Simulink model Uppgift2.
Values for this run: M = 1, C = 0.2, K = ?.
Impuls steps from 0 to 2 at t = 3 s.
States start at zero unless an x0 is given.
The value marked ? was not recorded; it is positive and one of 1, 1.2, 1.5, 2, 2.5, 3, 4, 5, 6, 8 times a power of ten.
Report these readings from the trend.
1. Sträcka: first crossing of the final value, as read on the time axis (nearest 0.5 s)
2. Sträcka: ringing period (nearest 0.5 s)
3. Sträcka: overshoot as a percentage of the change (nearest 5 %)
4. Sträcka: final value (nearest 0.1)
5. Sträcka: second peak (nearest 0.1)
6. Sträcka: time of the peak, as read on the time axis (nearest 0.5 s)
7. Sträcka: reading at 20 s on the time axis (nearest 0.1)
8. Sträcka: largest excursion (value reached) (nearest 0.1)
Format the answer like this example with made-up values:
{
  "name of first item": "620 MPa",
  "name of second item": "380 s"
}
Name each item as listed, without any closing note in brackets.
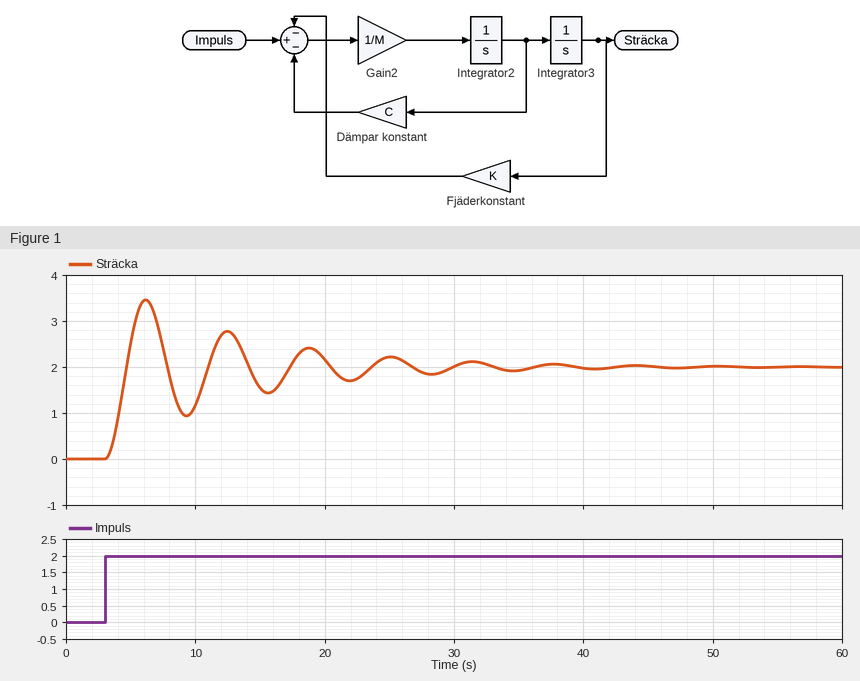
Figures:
{
  "Sträcka: first crossing of the final value, as read on the time axis": "4.5 s",
  "Sträcka: ringing period": "6.5 s",
  "Sträcka: overshoot as a percentage of the change": "75 %",
  "Sträcka: final value": "2.0",
  "Sträcka: second peak": "2.8",
  "Sträcka: time of the peak, as read on the time axis": "6.0 s",
  "Sträcka: reading at 20 s on the time axis": "2.2",
  "Sträcka: largest excursion (value reached)": "3.5"
}
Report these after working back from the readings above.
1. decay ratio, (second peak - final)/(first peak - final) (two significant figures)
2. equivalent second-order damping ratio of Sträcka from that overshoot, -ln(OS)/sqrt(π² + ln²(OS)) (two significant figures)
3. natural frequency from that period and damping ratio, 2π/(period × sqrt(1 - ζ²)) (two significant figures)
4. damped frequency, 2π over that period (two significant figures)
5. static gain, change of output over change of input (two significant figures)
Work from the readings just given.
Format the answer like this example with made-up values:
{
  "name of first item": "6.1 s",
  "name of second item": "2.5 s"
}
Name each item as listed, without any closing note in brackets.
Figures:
{
  "decay ratio, (second peak - final)/(first peak - final)": "0.53",
  "equivalent second-order damping ratio of Sträcka from that overshoot, -ln(OS)/sqrt(π² + ln²(OS))": "0.091",
  "natural frequency from that period and damping ratio, 2π/(period × sqrt(1 - ζ²))": "0.97 rad/s",
  "damped frequency, 2π over that period": "0.97 rad/s",
  "static gain, change of output over change of input": "1.0"
}
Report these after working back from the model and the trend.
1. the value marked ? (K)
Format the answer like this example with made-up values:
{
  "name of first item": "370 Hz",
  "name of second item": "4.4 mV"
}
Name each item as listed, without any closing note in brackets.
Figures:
{
  "the value marked ?": "1"
}
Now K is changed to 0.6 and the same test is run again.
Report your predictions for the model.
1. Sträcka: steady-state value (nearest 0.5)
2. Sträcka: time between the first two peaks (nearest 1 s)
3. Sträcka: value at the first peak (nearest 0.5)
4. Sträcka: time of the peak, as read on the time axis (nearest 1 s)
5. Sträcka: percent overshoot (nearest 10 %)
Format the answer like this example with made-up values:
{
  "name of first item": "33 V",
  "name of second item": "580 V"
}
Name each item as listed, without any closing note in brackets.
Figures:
{
  "Sträcka: steady-state value": "3.5",
  "Sträcka: time between the first two peaks": "8 s",
  "Sträcka: value at the first peak": "5.5",
  "Sträcka: time of the peak, as read on the time axis": "7 s",
  "Sträcka: percent overshoot": "70 %"
}
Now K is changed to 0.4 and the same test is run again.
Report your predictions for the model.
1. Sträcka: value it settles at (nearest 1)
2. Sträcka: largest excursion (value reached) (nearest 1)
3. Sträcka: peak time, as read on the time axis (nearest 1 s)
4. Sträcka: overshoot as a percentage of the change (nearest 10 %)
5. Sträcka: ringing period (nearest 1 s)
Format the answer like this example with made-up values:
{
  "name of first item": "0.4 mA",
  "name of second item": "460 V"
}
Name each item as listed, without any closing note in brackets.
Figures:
{
  "Sträcka: value it settles at": "5",
  "Sträcka: largest excursion (value reached)": "8",
  "Sträcka: peak time, as read on the time axis": "8 s",
  "Sträcka: overshoot as a percentage of the change": "60 %",
  "Sträcka: ringing period": "10 s"
}
